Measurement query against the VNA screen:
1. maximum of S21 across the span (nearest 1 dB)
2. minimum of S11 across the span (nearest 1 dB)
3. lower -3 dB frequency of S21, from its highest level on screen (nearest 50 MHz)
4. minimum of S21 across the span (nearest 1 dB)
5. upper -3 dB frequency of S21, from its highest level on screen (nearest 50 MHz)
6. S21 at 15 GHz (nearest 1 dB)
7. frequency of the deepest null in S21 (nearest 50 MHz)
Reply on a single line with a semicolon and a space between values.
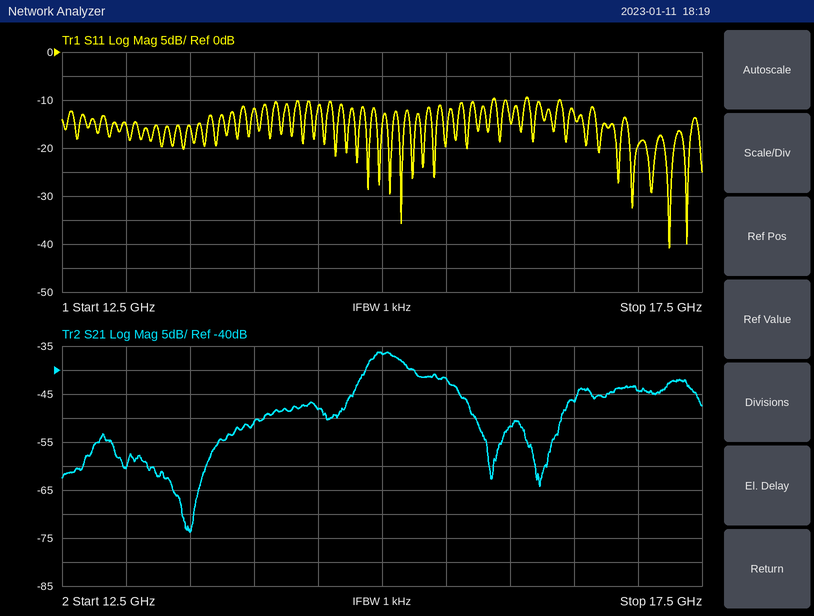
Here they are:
-36 dB; -41 dB; 14.90 GHz; -74 dB; 15.20 GHz; -37 dB; 13.50 GHz
